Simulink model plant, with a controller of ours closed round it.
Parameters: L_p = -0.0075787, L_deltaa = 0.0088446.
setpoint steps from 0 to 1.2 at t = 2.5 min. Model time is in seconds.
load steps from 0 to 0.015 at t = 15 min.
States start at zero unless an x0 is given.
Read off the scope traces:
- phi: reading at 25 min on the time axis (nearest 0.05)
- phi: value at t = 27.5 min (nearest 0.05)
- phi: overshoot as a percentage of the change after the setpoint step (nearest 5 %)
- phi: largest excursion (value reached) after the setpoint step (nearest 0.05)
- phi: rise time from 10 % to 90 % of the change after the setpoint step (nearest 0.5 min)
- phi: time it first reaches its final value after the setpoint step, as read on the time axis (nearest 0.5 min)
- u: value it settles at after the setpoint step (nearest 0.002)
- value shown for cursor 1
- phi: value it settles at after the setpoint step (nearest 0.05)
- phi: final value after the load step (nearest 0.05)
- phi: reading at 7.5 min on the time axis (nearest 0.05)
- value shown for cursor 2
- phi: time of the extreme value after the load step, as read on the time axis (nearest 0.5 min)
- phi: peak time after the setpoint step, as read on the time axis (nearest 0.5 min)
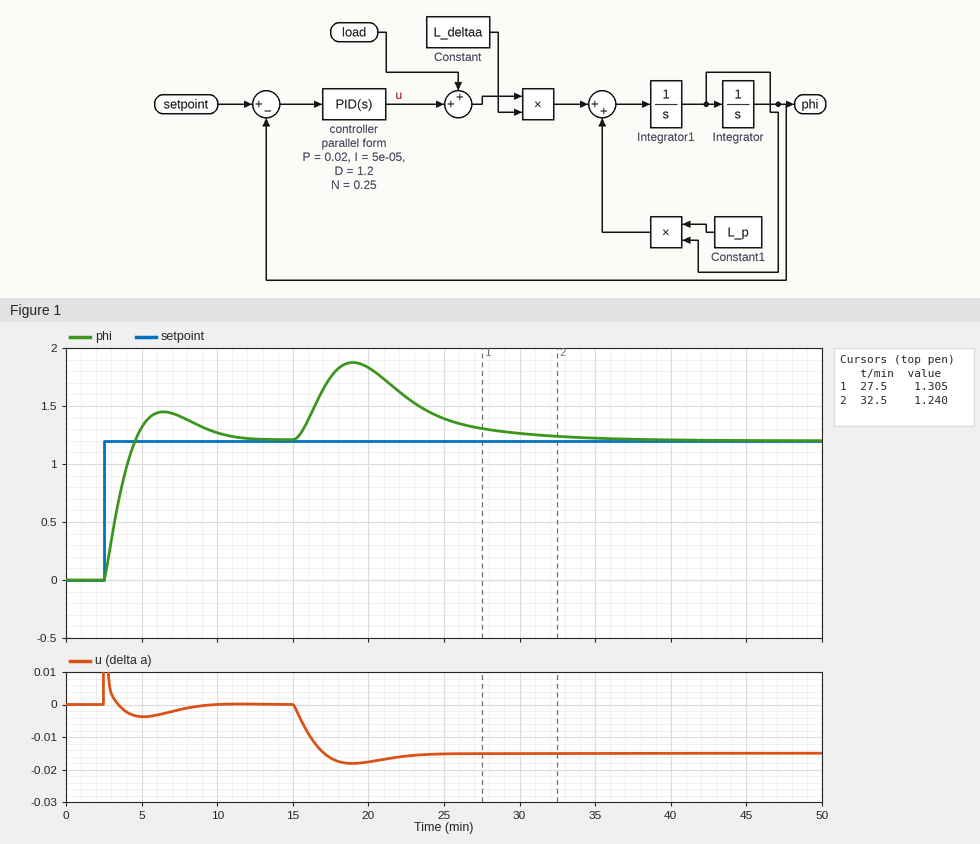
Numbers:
1.40
1.30
20 %
1.45
1.5 min
4.5 min
0.000
1.305
1.20
1.20
1.40
1.240
19.0 min
6.5 min
